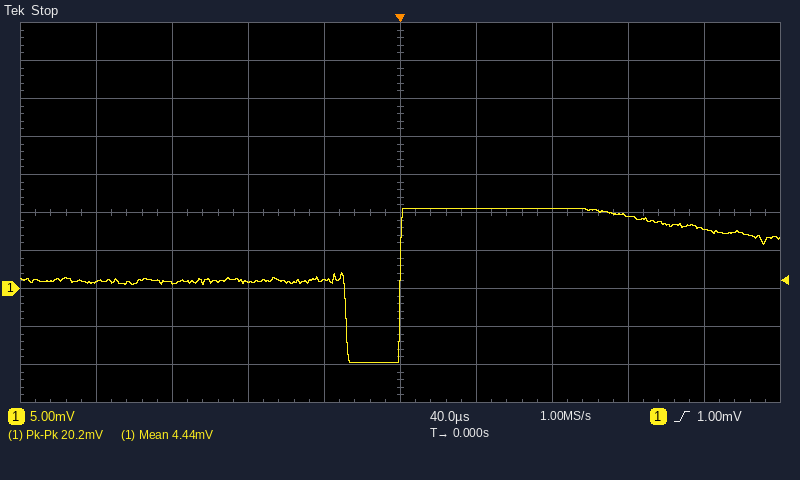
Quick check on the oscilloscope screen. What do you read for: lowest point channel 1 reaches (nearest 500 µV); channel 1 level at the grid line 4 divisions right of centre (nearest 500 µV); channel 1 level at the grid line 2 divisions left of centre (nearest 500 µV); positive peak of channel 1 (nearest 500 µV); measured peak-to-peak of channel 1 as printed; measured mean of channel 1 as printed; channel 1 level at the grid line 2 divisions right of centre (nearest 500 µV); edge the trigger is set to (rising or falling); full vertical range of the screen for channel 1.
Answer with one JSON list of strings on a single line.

["-9.5 mV", "8.0 mV", "1.0 mV", "10.5 mV", "20.2 mV", "4.44 mV", "10.5 mV", "rising", "50 mV"]
